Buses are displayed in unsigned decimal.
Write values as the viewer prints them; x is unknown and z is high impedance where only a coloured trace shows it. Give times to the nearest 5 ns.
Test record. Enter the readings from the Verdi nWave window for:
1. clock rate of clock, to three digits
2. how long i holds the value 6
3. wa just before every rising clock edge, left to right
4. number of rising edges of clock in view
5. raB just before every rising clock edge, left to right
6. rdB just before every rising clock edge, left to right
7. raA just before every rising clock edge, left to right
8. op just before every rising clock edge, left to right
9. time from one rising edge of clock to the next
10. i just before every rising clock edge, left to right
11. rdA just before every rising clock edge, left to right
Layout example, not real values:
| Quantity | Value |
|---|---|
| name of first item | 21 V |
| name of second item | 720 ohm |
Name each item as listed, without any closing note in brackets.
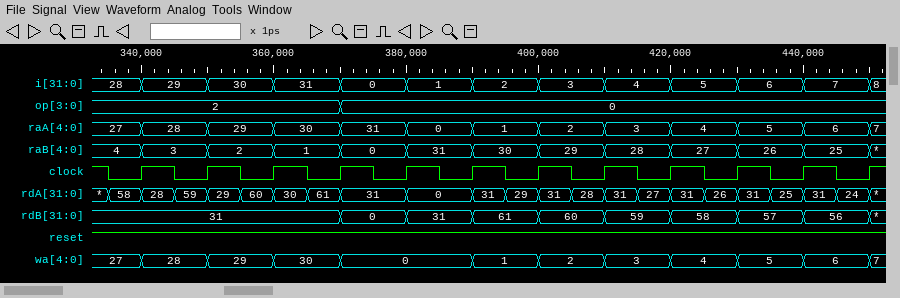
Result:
| Quantity | Value |
|---|---|
| clock rate of clock, to three digits | 100 MHz |
| how long i holds the value 6 | 10 ns |
| wa just before every rising clock edge, left to right | 27, 28, 29, 30, 0, 0, 1, 2, 3, 4, 5, 6 |
| number of rising edges of clock in view | 12 |
| raB just before every rising clock edge, left to right | 4, 3, 2, 1, 0, 31, 30, 29, 28, 27, 26, 25 |
| rdB just before every rising clock edge, left to right | 31, 31, 31, 31, 0, 31, 61, 60, 59, 58, 57, 56 |
| raA just before every rising clock edge, left to right | 27, 28, 29, 30, 31, 0, 1, 2, 3, 4, 5, 6 |
| op just before every rising clock edge, left to right | 2, 2, 2, 2, 0, 0, 0, 0, 0, 0, 0, 0 |
| time from one rising edge of clock to the next | 10 ns |
| i just before every rising clock edge, left to right | 28, 29, 30, 31, 0, 1, 2, 3, 4, 5, 6, 7 |
| rdA just before every rising clock edge, left to right | 58, 59, 60, 61, 31, 0, 29, 28, 27, 26, 25, 24 |
